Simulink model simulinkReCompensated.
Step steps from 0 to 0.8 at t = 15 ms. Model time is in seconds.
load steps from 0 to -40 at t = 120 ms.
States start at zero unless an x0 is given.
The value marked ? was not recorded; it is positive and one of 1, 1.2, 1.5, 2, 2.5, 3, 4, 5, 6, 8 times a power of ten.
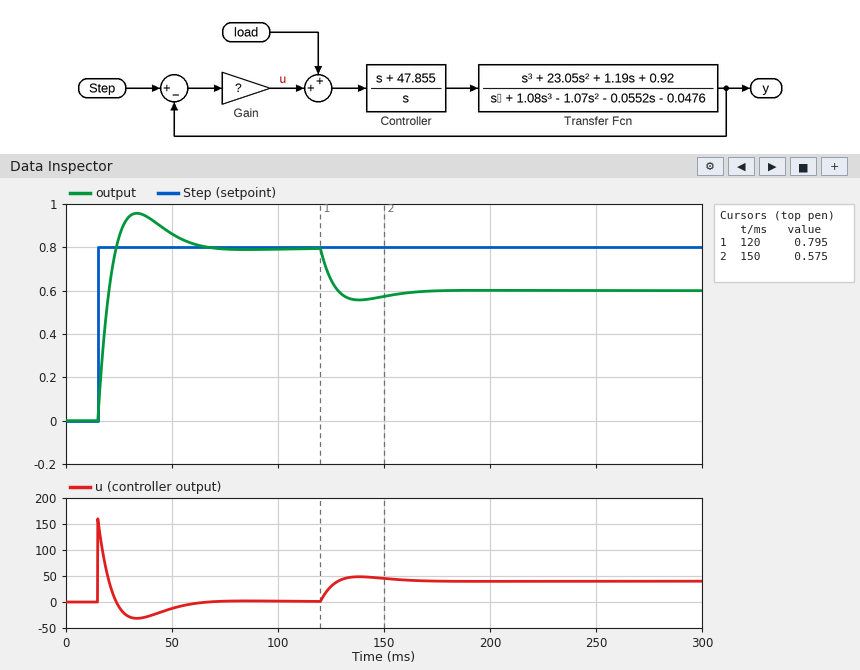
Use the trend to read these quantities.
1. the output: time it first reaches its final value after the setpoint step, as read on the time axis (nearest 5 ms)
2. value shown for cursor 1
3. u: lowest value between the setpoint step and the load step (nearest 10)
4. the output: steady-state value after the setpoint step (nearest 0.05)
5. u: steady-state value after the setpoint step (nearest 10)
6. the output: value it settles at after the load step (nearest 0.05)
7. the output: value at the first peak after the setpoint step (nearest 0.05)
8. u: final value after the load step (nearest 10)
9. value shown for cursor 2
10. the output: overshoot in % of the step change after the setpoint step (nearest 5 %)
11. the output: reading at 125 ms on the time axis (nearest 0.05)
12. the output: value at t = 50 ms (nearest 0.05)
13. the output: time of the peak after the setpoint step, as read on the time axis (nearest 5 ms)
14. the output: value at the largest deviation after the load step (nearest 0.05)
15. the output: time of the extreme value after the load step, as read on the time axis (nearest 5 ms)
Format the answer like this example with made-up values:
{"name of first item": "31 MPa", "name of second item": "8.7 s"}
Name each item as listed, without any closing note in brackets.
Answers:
{"the output: time it first reaches its final value after the setpoint step, as read on the time axis": "25 ms", "value shown for cursor 1": "0.795", "u: lowest value between the setpoint step and the load step": "-30", "the output: steady-state value after the setpoint step": "0.80", "u: steady-state value after the setpoint step": "0", "the output: value it settles at after the load step": "0.60", "the output: value at the first peak after the setpoint step": "0.95", "u: final value after the load step": "40", "value shown for cursor 2": "0.575", "the output: overshoot in % of the step change after the setpoint step": "20 %", "the output: reading at 125 ms on the time axis": "0.65", "the output: value at t = 50 ms": "0.85", "the output: time of the peak after the setpoint step, as read on the time axis": "35 ms", "the output: value at the largest deviation after the load step": "0.55", "the output: time of the extreme value after the load step, as read on the time axis": "140 ms"}
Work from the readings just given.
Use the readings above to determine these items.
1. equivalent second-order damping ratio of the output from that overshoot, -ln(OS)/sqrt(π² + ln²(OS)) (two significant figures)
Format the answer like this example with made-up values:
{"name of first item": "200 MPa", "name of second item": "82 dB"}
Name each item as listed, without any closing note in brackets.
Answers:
{"equivalent second-order damping ratio of the output from that overshoot, -ln(OS)/sqrt(π² + ln²(OS))": "0.46"}
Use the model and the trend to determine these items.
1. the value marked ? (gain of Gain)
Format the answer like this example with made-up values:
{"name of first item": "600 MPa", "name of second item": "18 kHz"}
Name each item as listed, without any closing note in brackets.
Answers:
{"the value marked ?": "200"}
